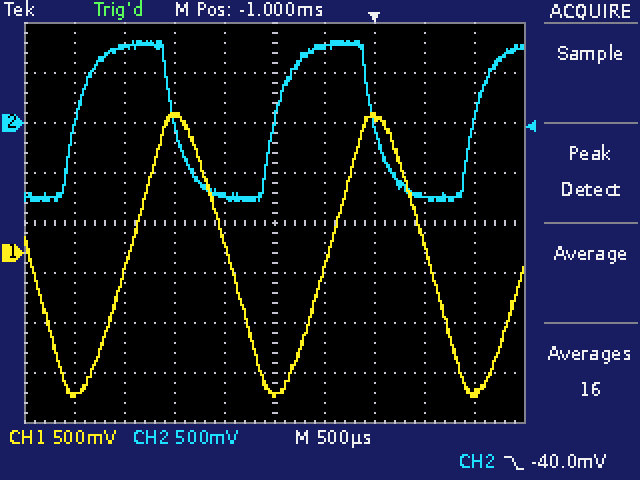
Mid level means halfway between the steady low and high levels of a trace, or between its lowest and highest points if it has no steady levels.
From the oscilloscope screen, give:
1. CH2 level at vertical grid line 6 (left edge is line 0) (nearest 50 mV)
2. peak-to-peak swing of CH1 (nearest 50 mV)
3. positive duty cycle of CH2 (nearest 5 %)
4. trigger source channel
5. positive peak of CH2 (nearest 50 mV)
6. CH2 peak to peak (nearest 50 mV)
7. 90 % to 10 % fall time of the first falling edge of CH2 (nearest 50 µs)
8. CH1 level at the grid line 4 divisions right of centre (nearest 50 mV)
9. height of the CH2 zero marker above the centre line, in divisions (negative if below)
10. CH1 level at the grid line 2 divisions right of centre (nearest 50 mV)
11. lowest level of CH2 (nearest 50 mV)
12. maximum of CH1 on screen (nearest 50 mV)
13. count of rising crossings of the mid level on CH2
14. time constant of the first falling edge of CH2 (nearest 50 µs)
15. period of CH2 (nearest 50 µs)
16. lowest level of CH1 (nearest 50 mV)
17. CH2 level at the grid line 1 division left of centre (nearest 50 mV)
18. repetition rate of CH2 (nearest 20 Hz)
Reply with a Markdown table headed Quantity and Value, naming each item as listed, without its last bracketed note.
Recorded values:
| Quantity | Value |
|---|---|
| CH2 level at vertical grid line 6 (left edge is line 0) | 750 mV |
| peak-to-peak swing of CH1 | 2.85 V |
| positive duty cycle of CH2 | 50 % |
| trigger source channel | CH2 |
| positive peak of CH2 | 800 mV |
| CH2 peak to peak | 1.60 V |
| 90 % to 10 % fall time of the first falling edge of CH2 | 350 µs |
| CH1 level at the grid line 4 divisions right of centre | -1.40 V |
| height of the CH2 zero marker above the centre line, in divisions | +2.0 div |
| CH1 level at the grid line 2 divisions right of centre | 1.35 V |
| lowest level of CH2 | -800 mV |
| maximum of CH1 on screen | 1.40 V |
| count of rising crossings of the mid level on CH2 | 3 |
| time constant of the first falling edge of CH2 | 150 µs |
| period of CH2 | 2.00 ms |
| lowest level of CH1 | -1.45 V |
| CH2 level at the grid line 1 division left of centre | -750 mV |
| repetition rate of CH2 | 500 Hz |
